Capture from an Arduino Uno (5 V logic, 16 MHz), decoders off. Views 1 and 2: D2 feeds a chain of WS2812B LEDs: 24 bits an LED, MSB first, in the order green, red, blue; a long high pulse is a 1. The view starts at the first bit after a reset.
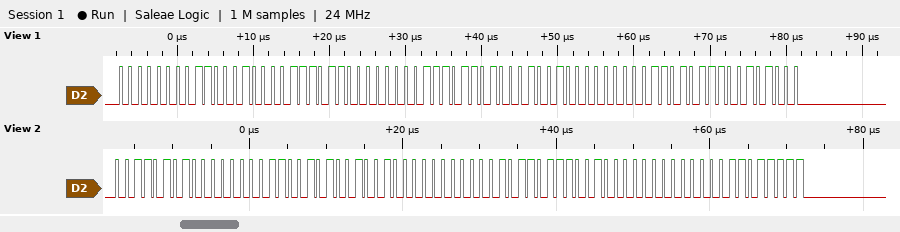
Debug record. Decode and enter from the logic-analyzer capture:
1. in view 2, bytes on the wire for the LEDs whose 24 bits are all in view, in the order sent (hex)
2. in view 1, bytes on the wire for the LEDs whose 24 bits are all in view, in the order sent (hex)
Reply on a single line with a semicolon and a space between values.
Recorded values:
35 00 CA 48 00 B7 20 00 DF; 00 C4 3B 00 ED 12 00 D7 28
